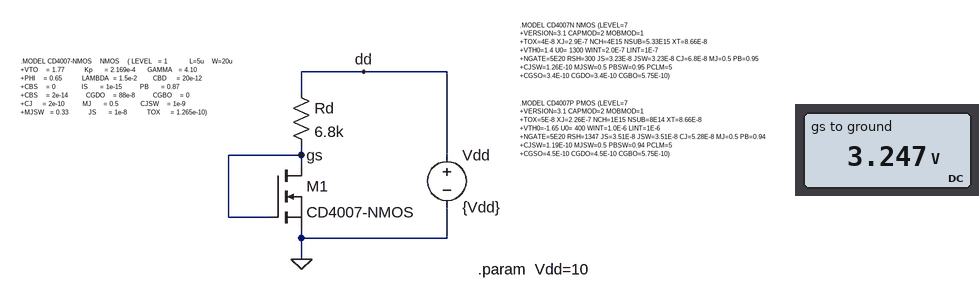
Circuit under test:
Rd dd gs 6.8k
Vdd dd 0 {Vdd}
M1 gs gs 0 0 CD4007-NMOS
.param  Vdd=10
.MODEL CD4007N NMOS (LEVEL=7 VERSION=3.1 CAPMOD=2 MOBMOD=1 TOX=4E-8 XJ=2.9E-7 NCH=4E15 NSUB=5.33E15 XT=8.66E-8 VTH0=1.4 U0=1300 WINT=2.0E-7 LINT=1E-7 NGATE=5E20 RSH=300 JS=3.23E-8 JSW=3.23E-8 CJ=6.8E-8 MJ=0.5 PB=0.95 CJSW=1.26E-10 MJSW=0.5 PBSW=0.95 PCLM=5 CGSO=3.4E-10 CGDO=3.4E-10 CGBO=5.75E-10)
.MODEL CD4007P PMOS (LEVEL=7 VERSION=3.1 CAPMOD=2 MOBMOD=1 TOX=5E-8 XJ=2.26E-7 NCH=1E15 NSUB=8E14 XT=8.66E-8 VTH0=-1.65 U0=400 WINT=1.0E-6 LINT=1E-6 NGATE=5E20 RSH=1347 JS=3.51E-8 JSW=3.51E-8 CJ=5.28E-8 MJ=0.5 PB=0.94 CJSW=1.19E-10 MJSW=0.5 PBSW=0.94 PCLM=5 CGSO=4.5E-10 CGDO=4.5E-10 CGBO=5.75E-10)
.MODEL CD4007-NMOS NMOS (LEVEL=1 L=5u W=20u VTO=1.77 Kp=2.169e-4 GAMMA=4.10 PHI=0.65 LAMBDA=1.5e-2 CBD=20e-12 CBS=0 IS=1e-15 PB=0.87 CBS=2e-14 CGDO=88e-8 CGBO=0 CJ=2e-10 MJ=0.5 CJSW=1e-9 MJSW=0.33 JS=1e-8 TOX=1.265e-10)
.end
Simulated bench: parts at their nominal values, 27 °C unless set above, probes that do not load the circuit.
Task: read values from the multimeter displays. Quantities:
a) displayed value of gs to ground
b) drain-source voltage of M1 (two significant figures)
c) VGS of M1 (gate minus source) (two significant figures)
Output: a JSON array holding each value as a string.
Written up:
["3.247 V", "3.2 V", "3.2 V"]
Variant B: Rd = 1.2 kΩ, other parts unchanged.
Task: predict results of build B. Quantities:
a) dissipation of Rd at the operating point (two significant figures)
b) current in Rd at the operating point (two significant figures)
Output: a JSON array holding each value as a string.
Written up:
["22 mW", "4.3 mA"]
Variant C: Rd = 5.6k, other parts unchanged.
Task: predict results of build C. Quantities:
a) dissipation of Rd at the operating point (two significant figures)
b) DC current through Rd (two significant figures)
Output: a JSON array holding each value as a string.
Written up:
["7.8 mW", "1.2 mA"]
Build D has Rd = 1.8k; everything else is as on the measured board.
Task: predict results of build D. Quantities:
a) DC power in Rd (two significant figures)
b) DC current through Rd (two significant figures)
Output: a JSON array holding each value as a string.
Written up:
["18 mW", "3.1 mA"]
